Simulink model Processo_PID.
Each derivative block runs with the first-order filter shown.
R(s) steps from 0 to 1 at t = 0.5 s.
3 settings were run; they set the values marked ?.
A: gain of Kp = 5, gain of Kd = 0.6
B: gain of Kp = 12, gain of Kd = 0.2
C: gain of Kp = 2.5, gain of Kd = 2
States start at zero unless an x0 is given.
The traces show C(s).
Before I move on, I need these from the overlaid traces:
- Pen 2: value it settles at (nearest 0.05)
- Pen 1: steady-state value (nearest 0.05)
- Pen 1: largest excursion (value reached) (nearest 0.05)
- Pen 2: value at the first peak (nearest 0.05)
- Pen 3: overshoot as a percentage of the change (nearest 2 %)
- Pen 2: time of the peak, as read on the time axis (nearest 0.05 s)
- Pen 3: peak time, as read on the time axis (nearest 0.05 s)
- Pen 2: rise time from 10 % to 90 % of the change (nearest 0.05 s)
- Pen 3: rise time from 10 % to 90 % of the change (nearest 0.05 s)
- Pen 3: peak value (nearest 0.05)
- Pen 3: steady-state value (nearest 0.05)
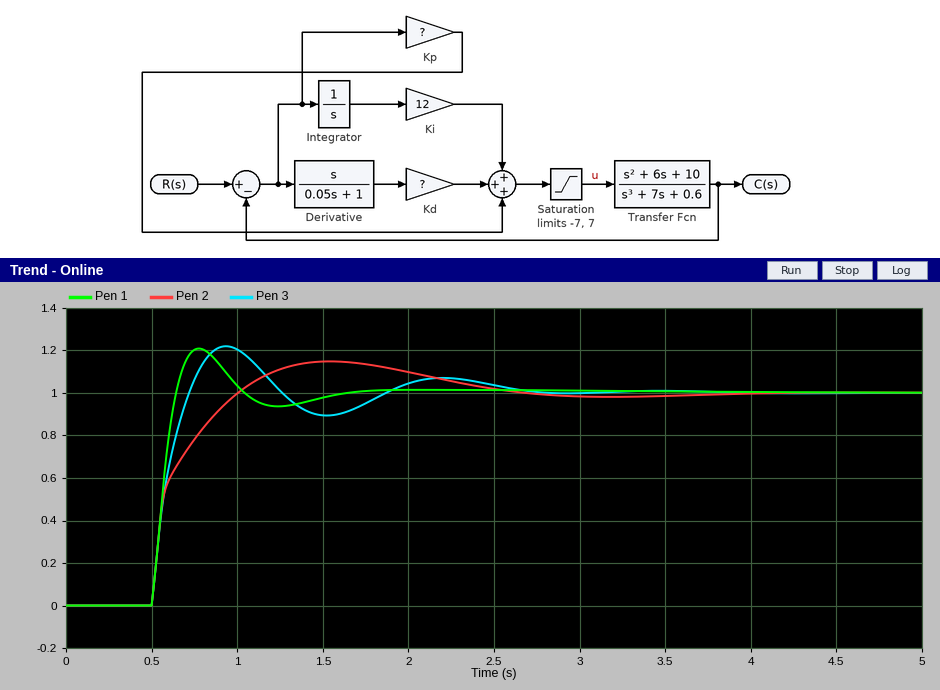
1.00
1.00
1.20
1.15
22 %
1.55 s
0.95 s
0.35 s
0.15 s
1.20
1.00
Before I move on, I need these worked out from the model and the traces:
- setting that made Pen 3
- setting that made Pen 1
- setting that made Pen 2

A
B
C
